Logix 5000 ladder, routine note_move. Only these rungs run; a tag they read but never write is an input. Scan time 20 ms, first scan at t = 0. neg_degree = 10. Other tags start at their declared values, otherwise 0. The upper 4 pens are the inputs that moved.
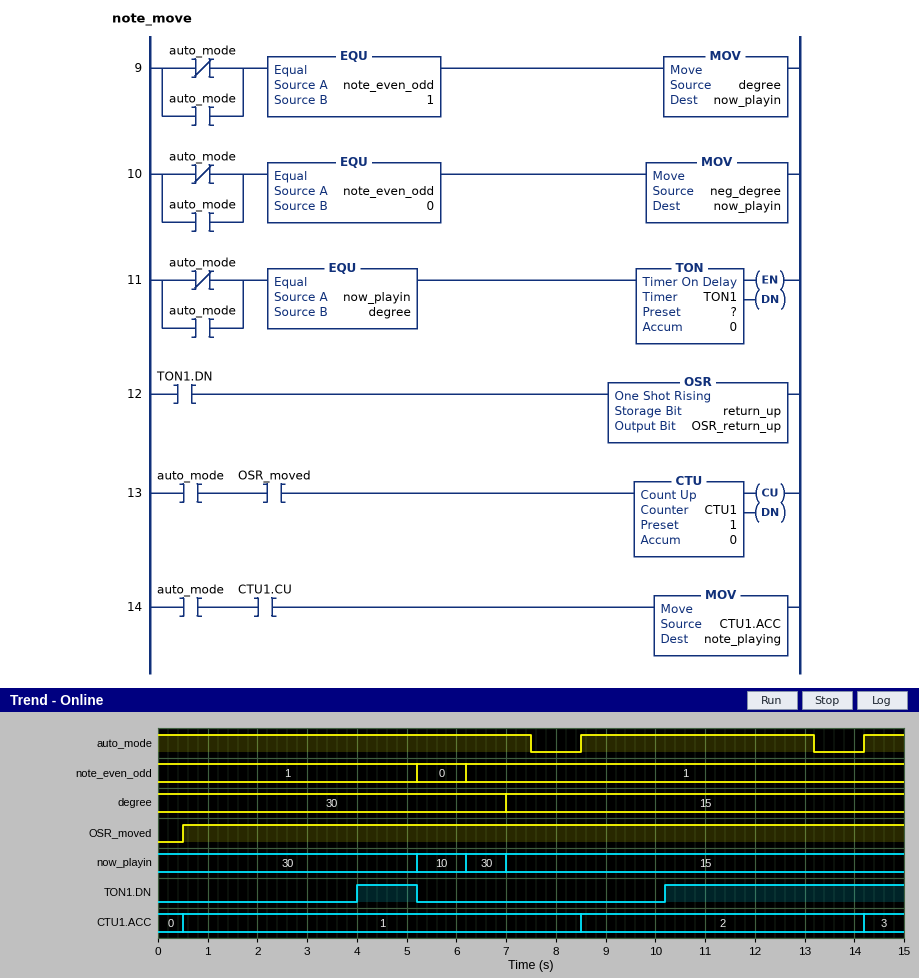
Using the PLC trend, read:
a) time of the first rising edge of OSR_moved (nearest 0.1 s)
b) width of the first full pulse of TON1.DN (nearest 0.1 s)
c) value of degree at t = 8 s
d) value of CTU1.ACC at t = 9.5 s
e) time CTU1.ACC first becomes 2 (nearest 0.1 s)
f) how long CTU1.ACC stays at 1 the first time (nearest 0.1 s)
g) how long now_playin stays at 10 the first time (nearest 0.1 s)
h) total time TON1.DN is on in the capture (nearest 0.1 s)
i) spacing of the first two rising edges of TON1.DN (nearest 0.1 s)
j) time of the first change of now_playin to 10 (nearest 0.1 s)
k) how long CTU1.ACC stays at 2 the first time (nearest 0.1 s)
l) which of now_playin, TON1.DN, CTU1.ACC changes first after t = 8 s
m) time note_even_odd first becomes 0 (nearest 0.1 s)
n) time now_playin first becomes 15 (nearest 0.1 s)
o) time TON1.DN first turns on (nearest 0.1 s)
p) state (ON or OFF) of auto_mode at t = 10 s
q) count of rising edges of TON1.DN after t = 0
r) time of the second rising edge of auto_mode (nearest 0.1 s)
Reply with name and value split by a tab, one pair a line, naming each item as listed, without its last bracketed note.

time of the first rising edge of OSR_moved	0.5 s
width of the first full pulse of TON1.DN	1.2 s
value of degree at t = 8 s	15
value of CTU1.ACC at t = 9.5 s	2
time CTU1.ACC first becomes 2	8.5 s
how long CTU1.ACC stays at 1 the first time	8.0 s
how long now_playin stays at 10 the first time	1.0 s
total time TON1.DN is on in the capture	6.0 s
spacing of the first two rising edges of TON1.DN	6.2 s
time of the first change of now_playin to 10	5.2 s
how long CTU1.ACC stays at 2 the first time	5.7 s
which of now_playin, TON1.DN, CTU1.ACC changes first after t = 8 s	CTU1.ACC
time note_even_odd first becomes 0	5.2 s
time now_playin first becomes 15	7.0 s
time TON1.DN first turns on	4.0 s
state (ON or OFF) of auto_mode at t = 10 s	ON
count of rising edges of TON1.DN after t = 0	2
time of the second rising edge of auto_mode	14.2 s
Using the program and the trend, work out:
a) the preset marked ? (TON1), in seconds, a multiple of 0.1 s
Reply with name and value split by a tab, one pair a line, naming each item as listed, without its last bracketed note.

the preset marked ? (TON1), in seconds, a multiple of 0.1 s	4.0 s
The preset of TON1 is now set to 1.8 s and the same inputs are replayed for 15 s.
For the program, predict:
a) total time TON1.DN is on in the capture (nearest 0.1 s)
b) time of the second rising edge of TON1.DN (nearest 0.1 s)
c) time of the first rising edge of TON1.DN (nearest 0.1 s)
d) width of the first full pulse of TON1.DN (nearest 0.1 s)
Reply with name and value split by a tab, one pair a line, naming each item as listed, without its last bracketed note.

total time TON1.DN is on in the capture	10.4 s
time of the second rising edge of TON1.DN	8.0 s
time of the first rising edge of TON1.DN	1.8 s
width of the first full pulse of TON1.DN	3.4 s
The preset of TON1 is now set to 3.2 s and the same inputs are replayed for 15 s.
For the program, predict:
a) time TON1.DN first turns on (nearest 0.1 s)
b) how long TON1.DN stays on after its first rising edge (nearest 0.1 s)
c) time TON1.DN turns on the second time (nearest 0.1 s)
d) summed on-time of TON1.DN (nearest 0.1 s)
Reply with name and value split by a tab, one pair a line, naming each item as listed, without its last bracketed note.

time TON1.DN first turns on	3.2 s
how long TON1.DN stays on after its first rising edge	2.0 s
time TON1.DN turns on the second time	9.4 s
summed on-time of TON1.DN	7.6 s
